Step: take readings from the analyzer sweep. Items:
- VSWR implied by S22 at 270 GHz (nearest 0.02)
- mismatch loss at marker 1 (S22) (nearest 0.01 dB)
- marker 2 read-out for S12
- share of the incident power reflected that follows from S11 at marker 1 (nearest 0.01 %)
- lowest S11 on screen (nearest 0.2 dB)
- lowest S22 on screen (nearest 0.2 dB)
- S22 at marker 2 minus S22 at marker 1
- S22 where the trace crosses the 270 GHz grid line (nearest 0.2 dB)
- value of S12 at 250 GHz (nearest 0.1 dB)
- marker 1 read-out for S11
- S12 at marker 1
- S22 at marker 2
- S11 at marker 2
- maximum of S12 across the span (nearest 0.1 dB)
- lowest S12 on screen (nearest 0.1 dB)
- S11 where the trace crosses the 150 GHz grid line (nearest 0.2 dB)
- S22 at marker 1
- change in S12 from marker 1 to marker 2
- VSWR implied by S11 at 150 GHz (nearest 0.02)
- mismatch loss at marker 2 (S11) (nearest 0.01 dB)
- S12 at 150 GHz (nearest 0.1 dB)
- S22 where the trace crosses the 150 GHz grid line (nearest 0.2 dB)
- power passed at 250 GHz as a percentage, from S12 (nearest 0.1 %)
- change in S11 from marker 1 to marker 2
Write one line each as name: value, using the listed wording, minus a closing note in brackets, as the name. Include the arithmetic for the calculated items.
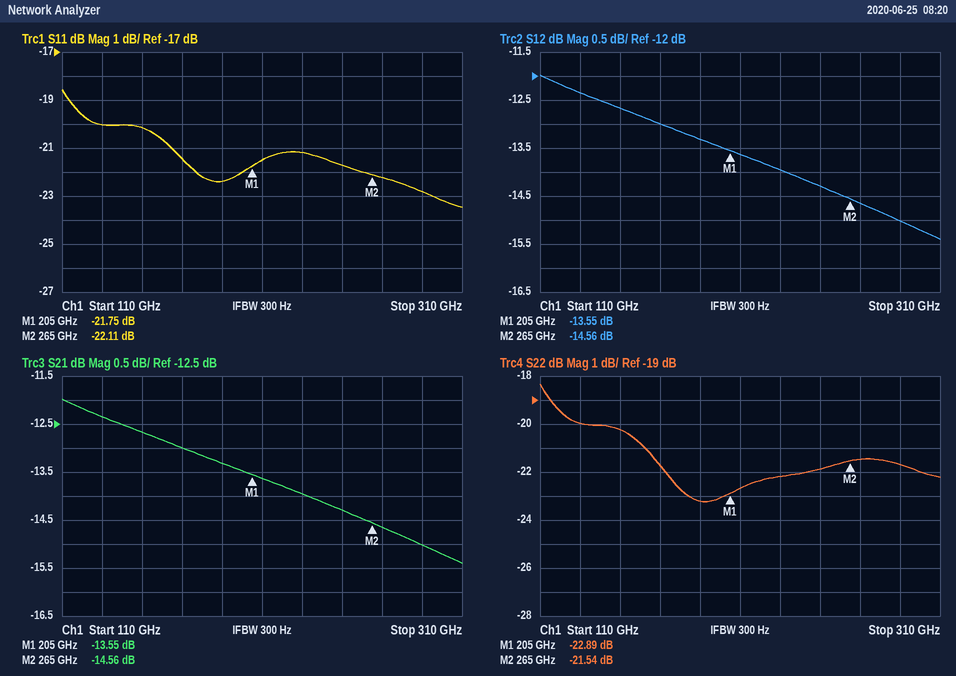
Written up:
VSWR implied by S22 at 270 GHz: |Γ| = 10^(-21.4/20) = 0.0851; VSWR = (1 + 0.0851)/(1 − 0.0851) ≈ 1.19, so 1.18 to the nearest 0.02
mismatch loss at marker 1 (S22): −10 log10(1 − 10^(-22.89/10)) ≈ 0.02 dB
marker 2 read-out for S12: -14.56 dB
share of the incident power reflected that follows from S11 at marker 1: 10^(-21.75/10) ≈ 0.67 %
lowest S11 on screen: -23.4 dB
lowest S22 on screen: -23.2 dB
S22 at marker 2 minus S22 at marker 1: -21.54 − (-22.89) = 1.35 dB
S22 where the trace crosses the 270 GHz grid line: -21.4 dB
value of S12 at 250 GHz: -14.3 dB
marker 1 read-out for S11: -21.75 dB
S12 at marker 1: -13.55 dB
S22 at marker 2: -21.54 dB
S11 at marker 2: -22.11 dB
maximum of S12 across the span: -12.0 dB
lowest S12 on screen: -15.4 dB
S11 where the trace crosses the 150 GHz grid line: -20.2 dB
S22 at marker 1: -22.89 dB
change in S12 from marker 1 to marker 2: -14.56 − (-13.55) = -1.01 dB
VSWR implied by S11 at 150 GHz: |Γ| = 10^(-20.2/20) = 0.0977; VSWR = (1 + 0.0977)/(1 − 0.0977) ≈ 1.22
mismatch loss at marker 2 (S11): −10 log10(1 − 10^(-22.11/10)) ≈ 0.03 dB
S12 at 150 GHz: -12.7 dB
S22 where the trace crosses the 150 GHz grid line: -20.2 dB
power passed at 250 GHz as a percentage, from S12: 10^(-14.3/10) ≈ 3.7 %
change in S11 from marker 1 to marker 2: -22.11 − (-21.75) = -0.36 dB
